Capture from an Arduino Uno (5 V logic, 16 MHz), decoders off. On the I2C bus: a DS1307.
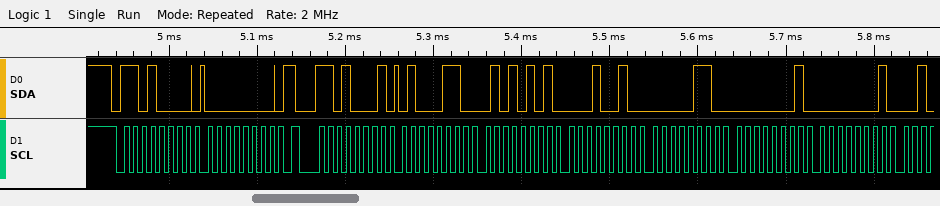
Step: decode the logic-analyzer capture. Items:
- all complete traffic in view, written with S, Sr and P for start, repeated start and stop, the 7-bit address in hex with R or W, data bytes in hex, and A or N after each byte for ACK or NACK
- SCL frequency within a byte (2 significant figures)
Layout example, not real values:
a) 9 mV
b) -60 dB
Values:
a) S 68W A 00 A Sr 68R A 46 A 55 A 12 A 06 A 01 A 01 A
b) 100 kHz
